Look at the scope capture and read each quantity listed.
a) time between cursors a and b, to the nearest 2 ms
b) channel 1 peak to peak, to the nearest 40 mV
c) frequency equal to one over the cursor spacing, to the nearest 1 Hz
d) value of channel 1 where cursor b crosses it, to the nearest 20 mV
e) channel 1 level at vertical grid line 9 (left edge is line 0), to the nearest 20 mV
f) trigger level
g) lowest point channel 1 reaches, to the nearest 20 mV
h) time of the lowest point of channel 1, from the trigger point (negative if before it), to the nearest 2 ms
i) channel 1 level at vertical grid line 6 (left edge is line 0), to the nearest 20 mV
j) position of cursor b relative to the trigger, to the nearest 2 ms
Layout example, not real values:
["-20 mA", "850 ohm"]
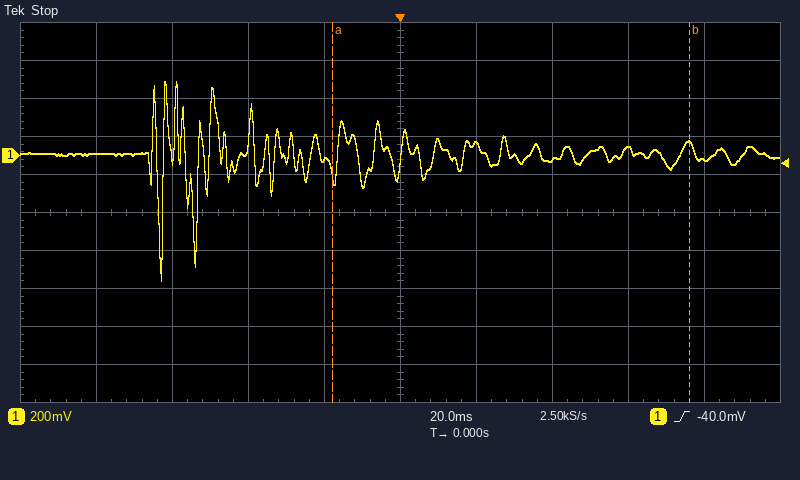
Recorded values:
["94 ms", "1.04 V", "11 Hz", "60 mV", "-20 mV", "-40.0 mV", "-660 mV", "-62 ms", "60 mV", "+76 ms"]
